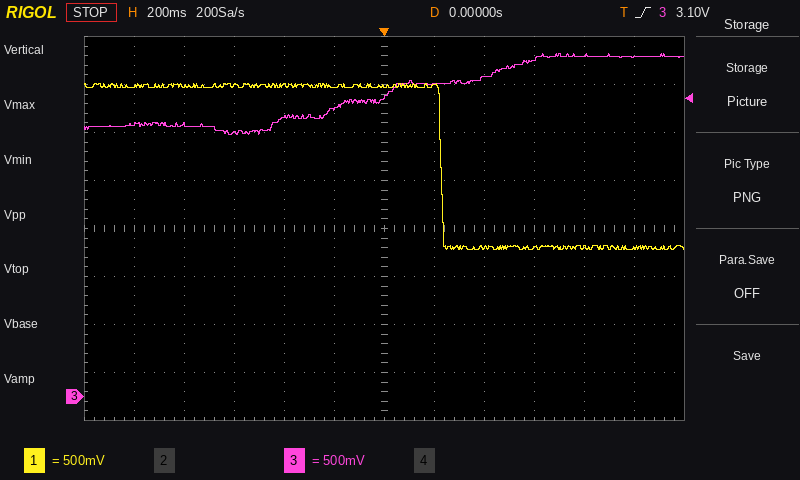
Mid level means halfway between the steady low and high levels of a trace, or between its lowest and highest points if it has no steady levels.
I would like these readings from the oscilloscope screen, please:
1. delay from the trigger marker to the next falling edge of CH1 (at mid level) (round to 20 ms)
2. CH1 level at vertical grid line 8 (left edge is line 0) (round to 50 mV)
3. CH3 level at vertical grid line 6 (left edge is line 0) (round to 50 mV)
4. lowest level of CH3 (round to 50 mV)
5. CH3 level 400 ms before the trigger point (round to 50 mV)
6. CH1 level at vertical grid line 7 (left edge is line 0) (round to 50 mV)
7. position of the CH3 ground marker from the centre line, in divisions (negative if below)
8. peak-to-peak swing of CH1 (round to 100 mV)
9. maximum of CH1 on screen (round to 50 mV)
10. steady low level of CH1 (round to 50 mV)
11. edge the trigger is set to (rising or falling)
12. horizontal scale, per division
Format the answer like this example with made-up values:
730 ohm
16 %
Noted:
220 ms
1.55 V
3.10 V
2.75 V
2.90 V
3.25 V
-3.5 div
1.70 V
3.25 V
1.55 V
rising
200 ms
